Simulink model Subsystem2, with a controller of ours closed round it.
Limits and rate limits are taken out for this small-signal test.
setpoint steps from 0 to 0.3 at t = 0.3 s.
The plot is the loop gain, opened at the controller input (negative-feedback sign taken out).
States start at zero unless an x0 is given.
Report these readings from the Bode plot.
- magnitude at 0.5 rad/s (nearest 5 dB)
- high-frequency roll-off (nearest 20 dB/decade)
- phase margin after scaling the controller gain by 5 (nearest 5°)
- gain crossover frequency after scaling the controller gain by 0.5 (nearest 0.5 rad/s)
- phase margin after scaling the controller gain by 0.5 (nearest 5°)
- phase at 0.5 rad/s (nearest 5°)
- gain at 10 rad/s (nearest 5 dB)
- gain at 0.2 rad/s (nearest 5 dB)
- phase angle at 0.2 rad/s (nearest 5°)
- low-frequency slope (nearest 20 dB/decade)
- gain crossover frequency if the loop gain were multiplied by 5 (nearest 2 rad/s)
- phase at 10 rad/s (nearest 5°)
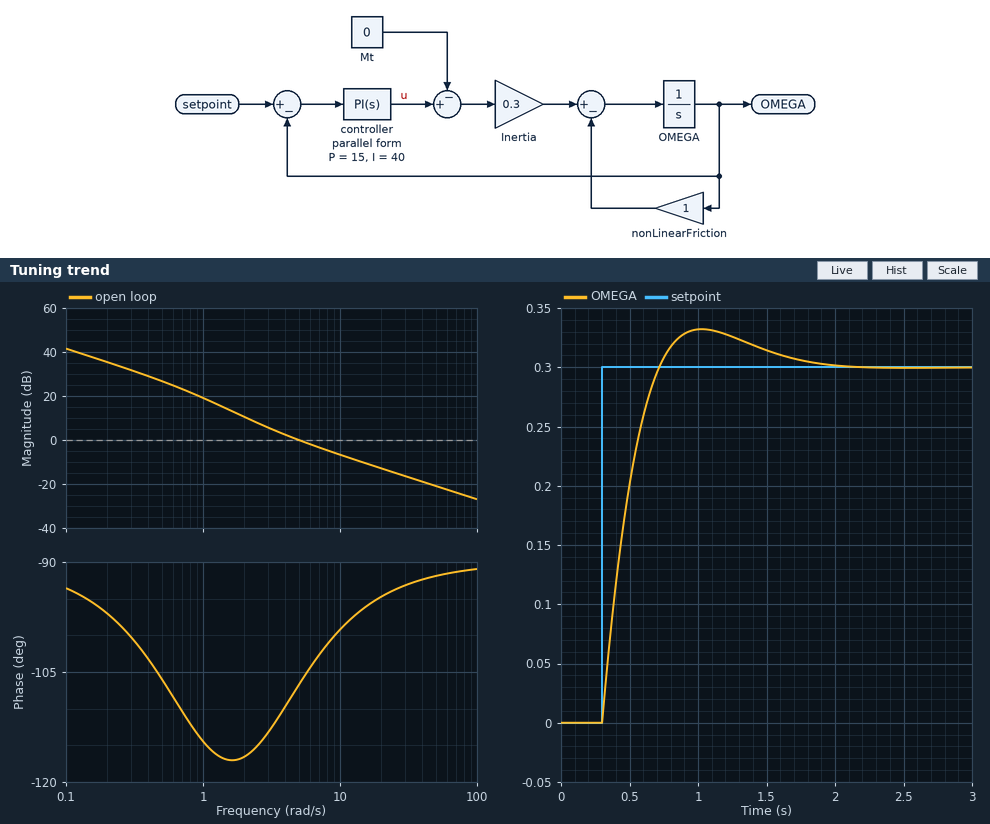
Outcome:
25 dB
-20 dB/decade
85°
3.0 rad/s
65°
-105°
-5 dB
35 dB
-95°
-20 dB/decade
22 rad/s
-100°
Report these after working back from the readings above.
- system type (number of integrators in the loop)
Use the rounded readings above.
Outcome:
1
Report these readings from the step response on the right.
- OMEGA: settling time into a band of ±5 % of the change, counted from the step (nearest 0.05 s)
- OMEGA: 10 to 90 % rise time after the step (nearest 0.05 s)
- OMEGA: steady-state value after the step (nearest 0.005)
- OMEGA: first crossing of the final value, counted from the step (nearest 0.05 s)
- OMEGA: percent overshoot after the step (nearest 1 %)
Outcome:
1.20 s
0.30 s
0.300
0.40 s
11 %
